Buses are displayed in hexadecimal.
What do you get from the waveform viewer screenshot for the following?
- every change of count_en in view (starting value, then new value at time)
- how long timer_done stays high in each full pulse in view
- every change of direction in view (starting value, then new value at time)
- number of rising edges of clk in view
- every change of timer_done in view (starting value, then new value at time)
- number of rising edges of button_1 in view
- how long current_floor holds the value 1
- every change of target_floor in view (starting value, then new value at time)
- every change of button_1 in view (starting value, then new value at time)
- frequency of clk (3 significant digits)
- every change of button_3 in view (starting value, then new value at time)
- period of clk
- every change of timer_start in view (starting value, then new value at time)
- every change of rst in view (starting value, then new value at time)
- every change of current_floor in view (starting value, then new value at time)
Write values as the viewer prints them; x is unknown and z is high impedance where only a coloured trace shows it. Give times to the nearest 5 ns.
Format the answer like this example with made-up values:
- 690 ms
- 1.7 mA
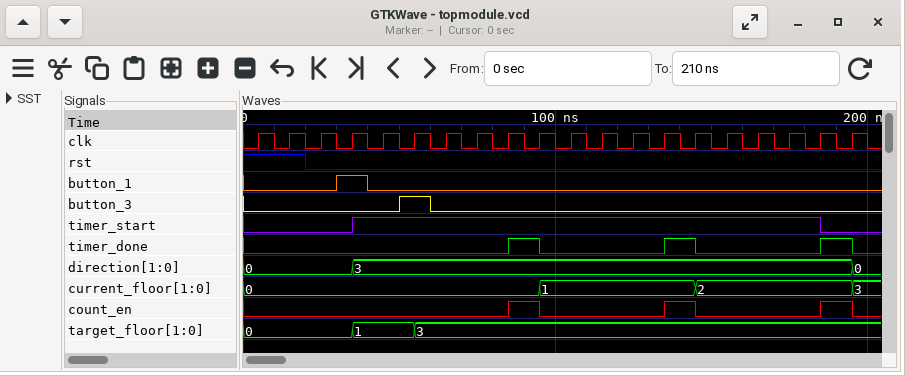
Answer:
- 0, 1 at 85 ns, 0 at 95 ns, 1 at 135 ns, 0 at 145 ns, 1 at 185 ns, 0 at 195 ns
- 10 ns, 10 ns, 10 ns
- 0, 3 at 35 ns, 0 at 195 ns
- 20
- 0, 1 at 85 ns, 0 at 95 ns, 1 at 135 ns, 0 at 145 ns, 1 at 185 ns, 0 at 195 ns
- 1
- 50 ns
- 0, 1 at 35 ns, 3 at 55 ns
- 0, 1 at 30 ns, 0 at 40 ns
- 100 MHz
- 0, 1 at 50 ns, 0 at 60 ns
- 10 ns
- 0, 1 at 35 ns, 0 at 185 ns
- 1, 0 at 20 ns
- 0, 1 at 95 ns, 2 at 145 ns, 3 at 195 ns
